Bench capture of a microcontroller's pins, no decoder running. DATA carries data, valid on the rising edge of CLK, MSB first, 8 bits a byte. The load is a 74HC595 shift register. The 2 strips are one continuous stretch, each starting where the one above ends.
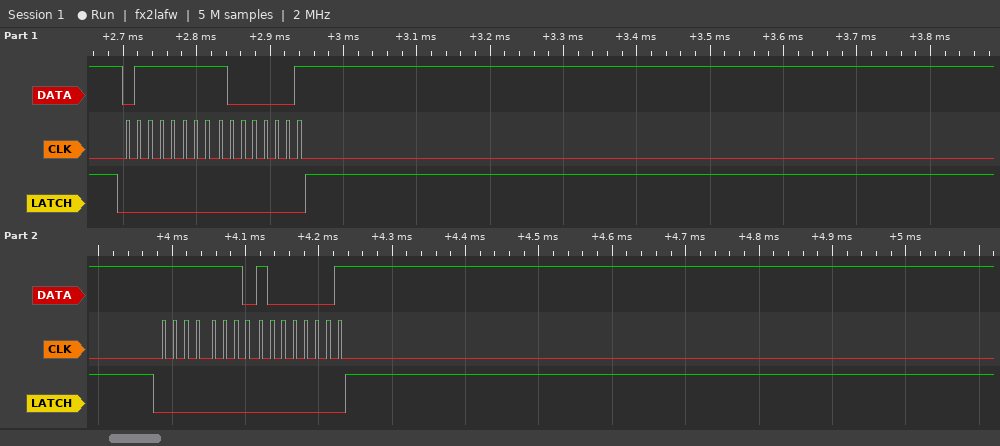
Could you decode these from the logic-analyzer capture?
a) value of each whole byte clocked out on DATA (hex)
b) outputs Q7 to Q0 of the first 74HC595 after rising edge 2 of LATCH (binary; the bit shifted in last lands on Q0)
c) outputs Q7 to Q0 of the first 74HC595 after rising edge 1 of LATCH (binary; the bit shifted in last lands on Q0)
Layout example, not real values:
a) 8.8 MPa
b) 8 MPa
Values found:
a) 7F 81 FE 81
b) 10000001
c) 10000001
